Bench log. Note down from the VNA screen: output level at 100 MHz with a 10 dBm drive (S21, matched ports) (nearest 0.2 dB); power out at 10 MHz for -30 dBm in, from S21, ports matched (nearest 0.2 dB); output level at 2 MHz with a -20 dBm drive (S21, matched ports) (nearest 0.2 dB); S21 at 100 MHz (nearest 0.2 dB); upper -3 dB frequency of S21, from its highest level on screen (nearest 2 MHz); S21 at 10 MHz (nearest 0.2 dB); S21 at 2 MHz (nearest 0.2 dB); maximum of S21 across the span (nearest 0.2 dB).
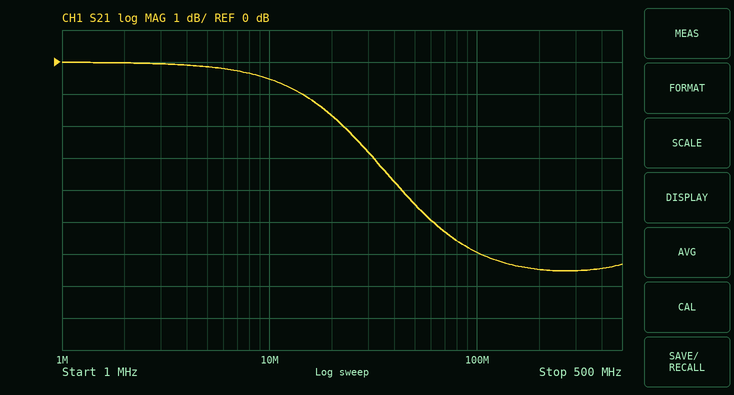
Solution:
4.0 dBm
-30.6 dBm
-20.0 dBm
-6.0 dB
32 MHz
-0.6 dB
0.0 dB
0.0 dB
